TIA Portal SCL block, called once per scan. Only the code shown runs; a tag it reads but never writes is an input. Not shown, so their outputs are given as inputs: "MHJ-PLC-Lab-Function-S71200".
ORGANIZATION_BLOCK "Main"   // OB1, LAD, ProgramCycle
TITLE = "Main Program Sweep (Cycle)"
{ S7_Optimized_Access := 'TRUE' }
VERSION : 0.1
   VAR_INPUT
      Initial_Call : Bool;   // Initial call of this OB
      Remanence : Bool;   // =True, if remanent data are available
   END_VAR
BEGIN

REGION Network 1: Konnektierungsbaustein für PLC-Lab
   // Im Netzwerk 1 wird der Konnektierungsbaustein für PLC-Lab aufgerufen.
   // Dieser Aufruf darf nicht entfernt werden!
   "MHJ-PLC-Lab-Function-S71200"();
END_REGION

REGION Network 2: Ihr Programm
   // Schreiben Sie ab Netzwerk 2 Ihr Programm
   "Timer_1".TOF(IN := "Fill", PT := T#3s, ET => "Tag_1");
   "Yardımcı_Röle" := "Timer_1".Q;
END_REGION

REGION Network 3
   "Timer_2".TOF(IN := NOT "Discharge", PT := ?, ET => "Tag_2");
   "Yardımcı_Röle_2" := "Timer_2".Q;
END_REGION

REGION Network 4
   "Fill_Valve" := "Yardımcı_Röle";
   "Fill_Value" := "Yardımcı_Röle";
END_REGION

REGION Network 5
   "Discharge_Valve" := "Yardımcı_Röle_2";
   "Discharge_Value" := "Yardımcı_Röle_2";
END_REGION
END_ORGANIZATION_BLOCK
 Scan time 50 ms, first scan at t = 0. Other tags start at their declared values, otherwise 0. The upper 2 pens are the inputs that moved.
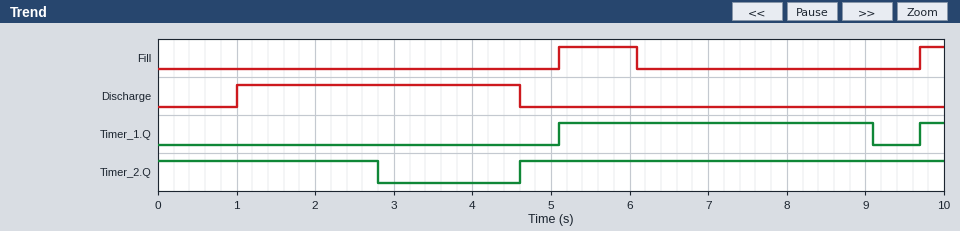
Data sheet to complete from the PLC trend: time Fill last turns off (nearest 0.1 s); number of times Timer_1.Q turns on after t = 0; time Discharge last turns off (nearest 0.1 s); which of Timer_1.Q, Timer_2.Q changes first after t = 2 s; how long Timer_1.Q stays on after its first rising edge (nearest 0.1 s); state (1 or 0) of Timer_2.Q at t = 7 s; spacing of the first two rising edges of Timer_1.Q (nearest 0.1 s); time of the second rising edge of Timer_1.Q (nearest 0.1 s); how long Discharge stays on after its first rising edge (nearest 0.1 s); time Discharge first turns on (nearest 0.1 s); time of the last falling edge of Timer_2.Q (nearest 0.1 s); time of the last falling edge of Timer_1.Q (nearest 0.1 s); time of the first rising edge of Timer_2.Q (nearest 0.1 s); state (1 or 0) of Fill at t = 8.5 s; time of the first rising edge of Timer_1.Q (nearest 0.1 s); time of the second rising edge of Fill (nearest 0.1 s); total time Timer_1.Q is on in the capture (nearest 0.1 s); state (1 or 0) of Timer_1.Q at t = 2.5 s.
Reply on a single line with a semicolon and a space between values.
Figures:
6.1 s; 2; 4.6 s; Timer_2.Q; 4.0 s; 1; 4.6 s; 9.7 s; 3.6 s; 1.0 s; 2.8 s; 9.1 s; 4.6 s; 0; 5.1 s; 9.7 s; 4.3 s; 0
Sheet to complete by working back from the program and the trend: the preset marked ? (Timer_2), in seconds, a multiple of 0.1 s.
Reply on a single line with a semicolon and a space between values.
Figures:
1.8 s
